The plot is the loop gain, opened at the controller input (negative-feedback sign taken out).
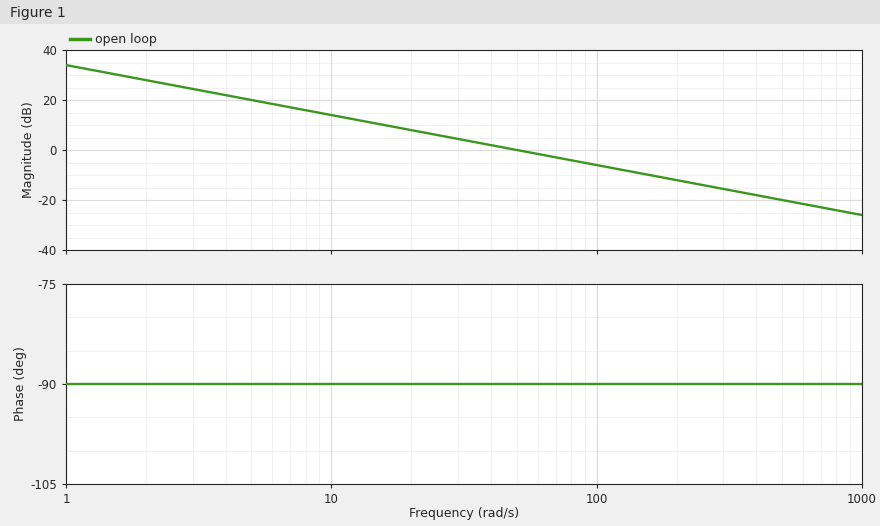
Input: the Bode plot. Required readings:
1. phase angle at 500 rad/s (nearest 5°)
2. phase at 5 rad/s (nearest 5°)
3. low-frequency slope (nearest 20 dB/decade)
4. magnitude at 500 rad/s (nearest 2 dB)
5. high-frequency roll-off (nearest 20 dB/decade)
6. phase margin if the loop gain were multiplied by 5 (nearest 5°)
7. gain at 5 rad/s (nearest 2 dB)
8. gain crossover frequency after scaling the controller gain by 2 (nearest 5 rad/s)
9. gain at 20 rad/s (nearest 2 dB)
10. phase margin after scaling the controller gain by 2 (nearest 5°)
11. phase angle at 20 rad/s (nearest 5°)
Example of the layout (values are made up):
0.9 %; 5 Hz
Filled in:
-90°; -90°; -20 dB/decade; -20 dB; -20 dB/decade; 90°; 20 dB; 100 rad/s; 8 dB; 90°; -90°
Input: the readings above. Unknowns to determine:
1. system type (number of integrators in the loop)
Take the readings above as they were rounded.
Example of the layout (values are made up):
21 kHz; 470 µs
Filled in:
1
